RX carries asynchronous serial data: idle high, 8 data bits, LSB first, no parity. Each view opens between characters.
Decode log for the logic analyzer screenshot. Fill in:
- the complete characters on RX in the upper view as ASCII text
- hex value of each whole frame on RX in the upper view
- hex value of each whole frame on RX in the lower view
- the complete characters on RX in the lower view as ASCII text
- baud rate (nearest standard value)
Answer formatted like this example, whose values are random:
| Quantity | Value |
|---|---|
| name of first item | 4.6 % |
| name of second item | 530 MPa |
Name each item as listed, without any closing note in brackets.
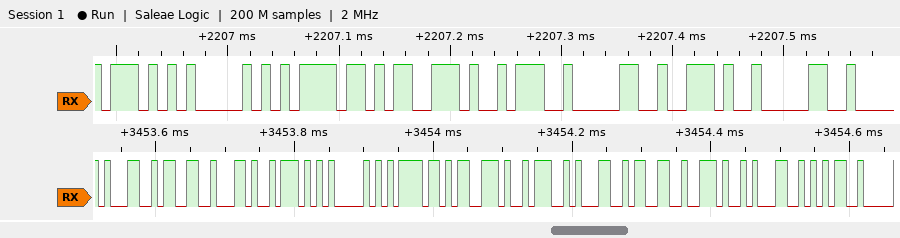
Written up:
| Quantity | Value |
|---|---|
| the complete characters on RX in the upper view as ASCII text | "WPos:0.0" |
| hex value of each whole frame on RX in the upper view | 57, 50, 6F, 73, 3A, 30, 2E, 30 |
| hex value of each whole frame on RX in the lower view | 31, 33, 2C, 57, 50, 6F, 73, 3A, 31, 33, 2E, 31, 35 |
| the complete characters on RX in the lower view as ASCII text | "13,WPos:13.15" |
| baud rate | 115200 baud |
